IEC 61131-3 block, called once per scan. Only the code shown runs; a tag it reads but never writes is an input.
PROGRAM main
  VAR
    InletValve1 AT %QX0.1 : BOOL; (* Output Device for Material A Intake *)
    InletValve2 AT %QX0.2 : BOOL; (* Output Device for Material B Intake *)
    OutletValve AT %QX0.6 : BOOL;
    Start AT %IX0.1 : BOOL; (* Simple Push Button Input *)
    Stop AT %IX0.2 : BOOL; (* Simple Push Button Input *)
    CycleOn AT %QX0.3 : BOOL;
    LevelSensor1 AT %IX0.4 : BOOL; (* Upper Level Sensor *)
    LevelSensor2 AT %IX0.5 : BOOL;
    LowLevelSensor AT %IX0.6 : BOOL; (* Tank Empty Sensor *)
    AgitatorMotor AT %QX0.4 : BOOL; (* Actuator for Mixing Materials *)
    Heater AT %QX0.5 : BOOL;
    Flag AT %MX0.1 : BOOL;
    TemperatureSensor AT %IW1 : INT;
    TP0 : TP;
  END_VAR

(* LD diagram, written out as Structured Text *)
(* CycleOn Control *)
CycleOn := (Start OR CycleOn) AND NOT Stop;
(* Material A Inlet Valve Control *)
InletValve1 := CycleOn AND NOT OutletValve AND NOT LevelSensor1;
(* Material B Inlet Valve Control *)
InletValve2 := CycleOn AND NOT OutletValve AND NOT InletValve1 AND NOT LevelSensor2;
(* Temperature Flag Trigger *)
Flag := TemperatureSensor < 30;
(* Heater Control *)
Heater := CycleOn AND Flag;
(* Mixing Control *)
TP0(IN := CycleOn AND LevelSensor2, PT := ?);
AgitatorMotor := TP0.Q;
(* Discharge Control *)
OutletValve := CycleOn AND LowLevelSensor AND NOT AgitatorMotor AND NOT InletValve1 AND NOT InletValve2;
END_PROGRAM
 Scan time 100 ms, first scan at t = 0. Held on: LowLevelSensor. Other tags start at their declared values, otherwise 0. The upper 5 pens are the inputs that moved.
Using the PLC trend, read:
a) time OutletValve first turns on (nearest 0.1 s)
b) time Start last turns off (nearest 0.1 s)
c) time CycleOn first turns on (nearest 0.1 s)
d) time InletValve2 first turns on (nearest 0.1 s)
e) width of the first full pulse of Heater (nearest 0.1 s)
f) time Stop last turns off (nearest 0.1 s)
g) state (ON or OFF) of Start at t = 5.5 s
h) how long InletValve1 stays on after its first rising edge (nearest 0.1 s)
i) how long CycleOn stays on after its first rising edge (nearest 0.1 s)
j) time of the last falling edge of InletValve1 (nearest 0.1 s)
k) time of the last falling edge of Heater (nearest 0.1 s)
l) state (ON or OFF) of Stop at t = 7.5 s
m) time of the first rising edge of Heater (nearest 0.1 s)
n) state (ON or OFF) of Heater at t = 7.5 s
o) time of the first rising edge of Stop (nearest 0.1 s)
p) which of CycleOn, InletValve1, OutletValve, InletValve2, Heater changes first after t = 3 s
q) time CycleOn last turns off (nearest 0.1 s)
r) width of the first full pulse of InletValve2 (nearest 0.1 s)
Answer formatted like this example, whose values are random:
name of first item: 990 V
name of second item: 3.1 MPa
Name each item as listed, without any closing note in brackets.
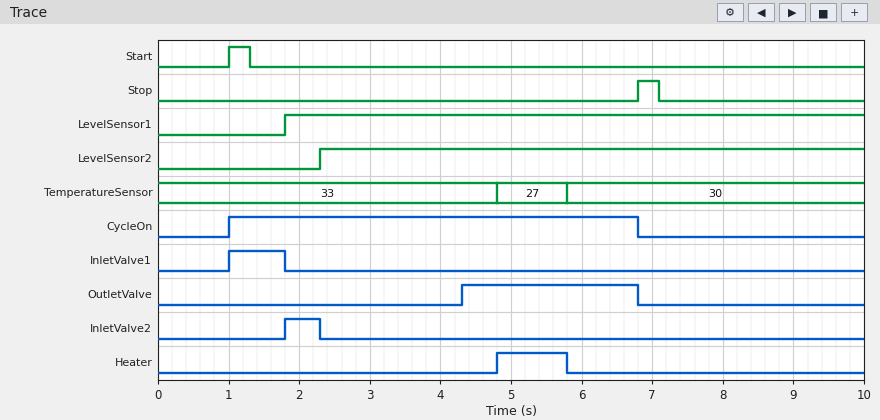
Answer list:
time OutletValve first turns on: 4.3 s
time Start last turns off: 1.3 s
time CycleOn first turns on: 1.0 s
time InletValve2 first turns on: 1.8 s
width of the first full pulse of Heater: 1.0 s
time Stop last turns off: 7.1 s
state (ON or OFF) of Start at t = 5.5 s: OFF
how long InletValve1 stays on after its first rising edge: 0.8 s
how long CycleOn stays on after its first rising edge: 5.8 s
time of the last falling edge of InletValve1: 1.8 s
time of the last falling edge of Heater: 5.8 s
state (ON or OFF) of Stop at t = 7.5 s: OFF
time of the first rising edge of Heater: 4.8 s
state (ON or OFF) of Heater at t = 7.5 s: OFF
time of the first rising edge of Stop: 6.8 s
which of CycleOn, InletValve1, OutletValve, InletValve2, Heater changes first after t = 3 s: OutletValve
time CycleOn last turns off: 6.8 s
width of the first full pulse of InletValve2: 0.5 s
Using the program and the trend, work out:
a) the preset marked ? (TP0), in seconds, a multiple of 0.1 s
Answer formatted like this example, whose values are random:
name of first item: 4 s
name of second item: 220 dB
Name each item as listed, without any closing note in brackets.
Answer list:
the preset marked ? (TP0), in seconds, a multiple of 0.1 s: 2.0 s
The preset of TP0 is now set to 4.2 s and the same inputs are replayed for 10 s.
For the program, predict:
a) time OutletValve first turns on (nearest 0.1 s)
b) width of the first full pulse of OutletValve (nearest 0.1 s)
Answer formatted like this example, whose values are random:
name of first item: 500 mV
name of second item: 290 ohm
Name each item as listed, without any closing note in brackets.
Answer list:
time OutletValve first turns on: 6.5 s
width of the first full pulse of OutletValve: 0.3 s
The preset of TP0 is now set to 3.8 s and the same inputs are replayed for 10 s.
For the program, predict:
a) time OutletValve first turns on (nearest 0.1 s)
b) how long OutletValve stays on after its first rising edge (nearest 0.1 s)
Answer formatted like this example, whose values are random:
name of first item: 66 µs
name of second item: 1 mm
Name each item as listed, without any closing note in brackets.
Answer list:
time OutletValve first turns on: 6.1 s
how long OutletValve stays on after its first rising edge: 0.7 s
